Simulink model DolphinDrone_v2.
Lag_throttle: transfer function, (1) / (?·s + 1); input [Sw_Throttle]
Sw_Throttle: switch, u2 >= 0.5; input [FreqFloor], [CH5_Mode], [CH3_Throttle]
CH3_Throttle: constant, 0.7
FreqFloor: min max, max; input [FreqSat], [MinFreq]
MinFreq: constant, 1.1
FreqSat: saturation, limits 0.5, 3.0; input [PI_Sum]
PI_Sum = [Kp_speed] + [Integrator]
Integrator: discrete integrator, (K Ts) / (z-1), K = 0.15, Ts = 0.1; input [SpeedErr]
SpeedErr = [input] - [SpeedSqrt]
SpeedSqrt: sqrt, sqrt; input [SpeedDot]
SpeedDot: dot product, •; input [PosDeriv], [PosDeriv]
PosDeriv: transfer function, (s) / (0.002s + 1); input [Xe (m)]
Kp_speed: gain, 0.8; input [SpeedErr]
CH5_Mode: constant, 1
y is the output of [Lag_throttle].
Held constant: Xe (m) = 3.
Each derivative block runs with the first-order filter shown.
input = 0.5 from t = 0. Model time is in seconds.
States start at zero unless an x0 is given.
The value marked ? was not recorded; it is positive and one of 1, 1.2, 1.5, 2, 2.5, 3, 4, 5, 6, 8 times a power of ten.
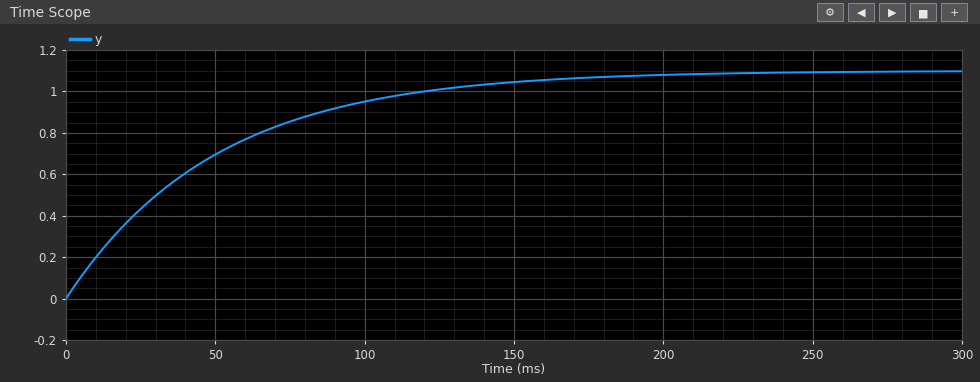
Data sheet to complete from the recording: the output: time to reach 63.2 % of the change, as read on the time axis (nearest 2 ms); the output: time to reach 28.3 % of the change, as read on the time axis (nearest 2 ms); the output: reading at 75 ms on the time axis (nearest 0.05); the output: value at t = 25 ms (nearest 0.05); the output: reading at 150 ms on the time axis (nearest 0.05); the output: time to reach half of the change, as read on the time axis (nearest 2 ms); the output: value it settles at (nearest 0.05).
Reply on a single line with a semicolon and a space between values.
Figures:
50 ms; 16 ms; 0.85; 0.45; 1.05; 34 ms; 1.10
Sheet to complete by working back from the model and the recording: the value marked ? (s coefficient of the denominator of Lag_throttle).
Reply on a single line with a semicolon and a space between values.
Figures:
0.05
